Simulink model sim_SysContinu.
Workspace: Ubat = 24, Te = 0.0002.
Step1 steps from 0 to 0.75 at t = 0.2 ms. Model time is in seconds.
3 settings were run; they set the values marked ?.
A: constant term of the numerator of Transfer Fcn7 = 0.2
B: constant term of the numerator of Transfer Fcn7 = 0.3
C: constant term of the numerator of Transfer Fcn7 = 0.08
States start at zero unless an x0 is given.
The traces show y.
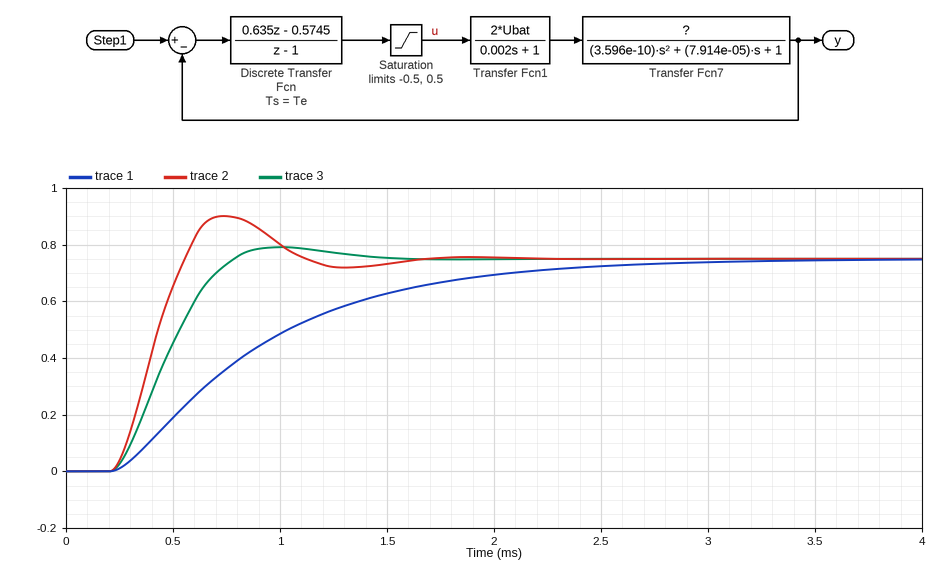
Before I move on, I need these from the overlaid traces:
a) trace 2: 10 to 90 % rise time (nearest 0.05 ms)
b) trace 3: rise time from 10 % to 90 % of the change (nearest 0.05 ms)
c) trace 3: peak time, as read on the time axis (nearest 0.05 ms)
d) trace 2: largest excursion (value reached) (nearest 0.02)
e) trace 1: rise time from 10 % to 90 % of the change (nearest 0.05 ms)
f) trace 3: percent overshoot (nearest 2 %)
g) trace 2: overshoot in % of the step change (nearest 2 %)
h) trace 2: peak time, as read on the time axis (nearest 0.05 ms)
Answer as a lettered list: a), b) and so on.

a) 0.25 ms
b) 0.40 ms
c) 1.00 ms
d) 0.90
e) 1.45 ms
f) 6 %
g) 20 %
h) 0.75 ms
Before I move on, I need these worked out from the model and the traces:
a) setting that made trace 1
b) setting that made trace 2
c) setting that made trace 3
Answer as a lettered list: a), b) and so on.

a) C
b) B
c) A
